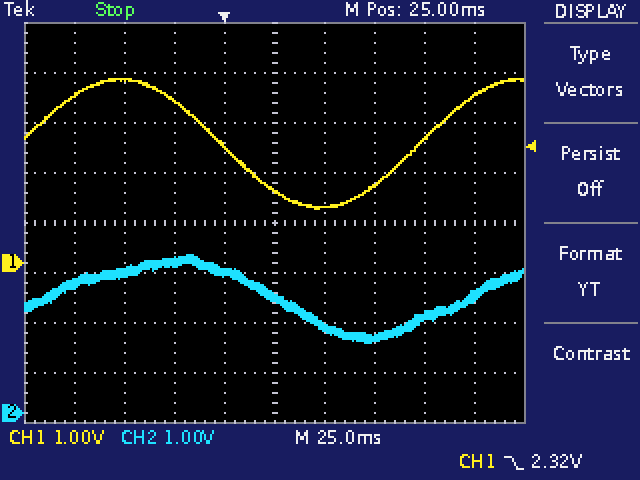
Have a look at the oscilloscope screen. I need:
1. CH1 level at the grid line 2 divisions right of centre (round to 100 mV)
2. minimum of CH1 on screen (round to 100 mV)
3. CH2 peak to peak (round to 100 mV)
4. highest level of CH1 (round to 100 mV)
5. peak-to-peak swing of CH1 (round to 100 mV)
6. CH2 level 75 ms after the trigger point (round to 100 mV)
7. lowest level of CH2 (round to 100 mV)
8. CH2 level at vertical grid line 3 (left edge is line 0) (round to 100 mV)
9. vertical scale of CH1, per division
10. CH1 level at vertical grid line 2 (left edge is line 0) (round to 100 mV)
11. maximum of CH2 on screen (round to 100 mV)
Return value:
1.5 V
1.1 V
1.8 V
3.7 V
2.6 V
1.5 V
1.4 V
3.0 V
1 V
3.7 V
3.2 V
